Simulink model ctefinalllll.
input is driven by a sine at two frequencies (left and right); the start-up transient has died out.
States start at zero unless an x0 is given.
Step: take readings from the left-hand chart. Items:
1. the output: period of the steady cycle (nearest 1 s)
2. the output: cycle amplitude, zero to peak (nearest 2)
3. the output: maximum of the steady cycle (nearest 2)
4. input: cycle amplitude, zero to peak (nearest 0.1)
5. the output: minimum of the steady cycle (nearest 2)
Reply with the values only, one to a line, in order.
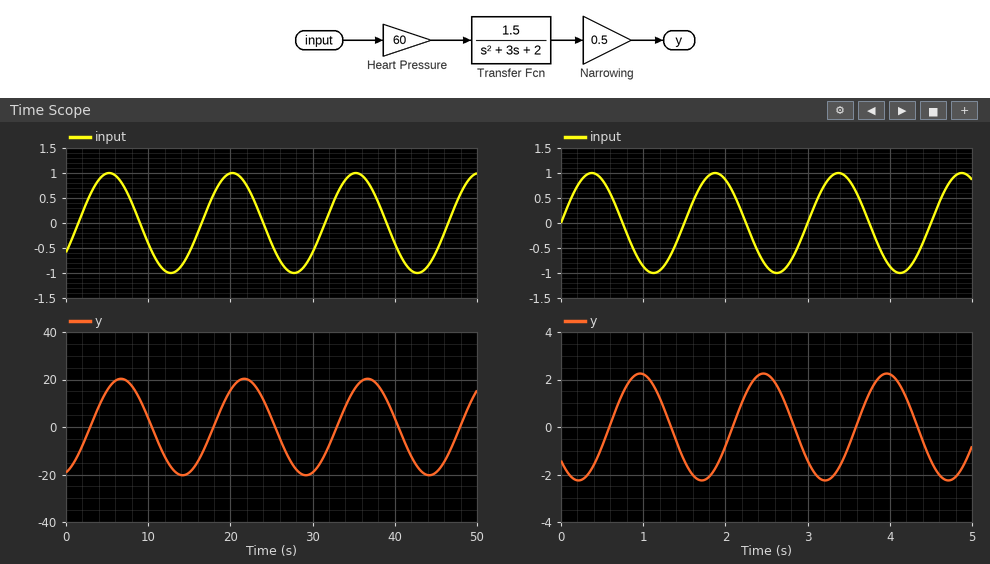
15 s
20
20
1.0
-20
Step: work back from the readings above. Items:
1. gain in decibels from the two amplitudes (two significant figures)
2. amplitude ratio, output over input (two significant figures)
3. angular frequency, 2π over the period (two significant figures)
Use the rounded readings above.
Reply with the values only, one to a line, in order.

26 dB
20
0.42 rad/s
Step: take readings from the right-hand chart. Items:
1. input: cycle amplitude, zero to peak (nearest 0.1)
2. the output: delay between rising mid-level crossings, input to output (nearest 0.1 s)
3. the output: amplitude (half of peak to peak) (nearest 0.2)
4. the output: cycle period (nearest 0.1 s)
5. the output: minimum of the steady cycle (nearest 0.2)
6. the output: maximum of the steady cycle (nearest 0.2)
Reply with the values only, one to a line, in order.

1.0
0.6 s
2.2
1.5 s
-2.2
2.2
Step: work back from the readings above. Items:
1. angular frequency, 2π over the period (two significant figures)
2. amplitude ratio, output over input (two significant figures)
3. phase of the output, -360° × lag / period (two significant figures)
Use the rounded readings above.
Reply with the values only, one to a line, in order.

4.2 rad/s
2.2
-140°
